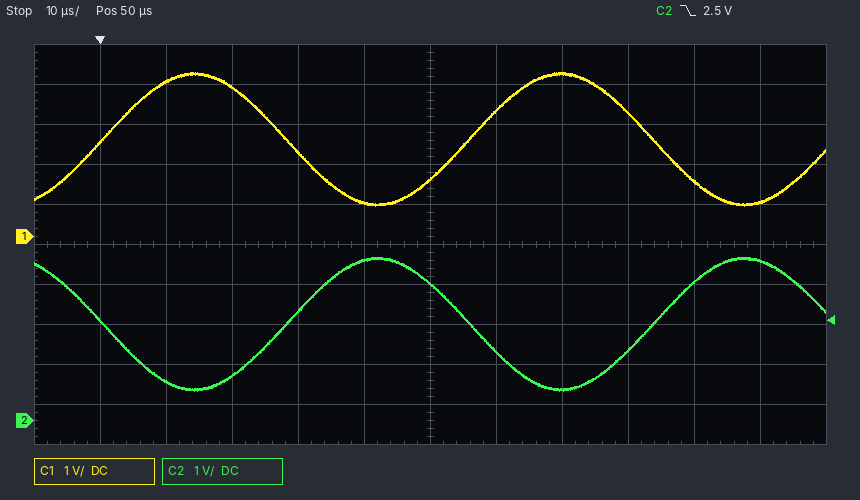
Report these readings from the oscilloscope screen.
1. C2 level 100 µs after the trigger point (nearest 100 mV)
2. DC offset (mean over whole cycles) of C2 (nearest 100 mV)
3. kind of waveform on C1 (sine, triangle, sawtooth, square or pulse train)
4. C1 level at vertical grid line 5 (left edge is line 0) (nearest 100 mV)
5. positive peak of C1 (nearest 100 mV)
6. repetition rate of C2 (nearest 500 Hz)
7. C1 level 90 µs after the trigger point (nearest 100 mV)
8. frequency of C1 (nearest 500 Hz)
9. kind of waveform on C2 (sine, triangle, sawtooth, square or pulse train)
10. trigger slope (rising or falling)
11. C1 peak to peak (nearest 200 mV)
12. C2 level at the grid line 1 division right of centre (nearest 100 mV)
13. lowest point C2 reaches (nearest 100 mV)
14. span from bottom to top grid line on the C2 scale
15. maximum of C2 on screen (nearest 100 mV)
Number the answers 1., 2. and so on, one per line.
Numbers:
1. 4.0 V
2. 2.4 V
3. sine
4. 800 mV
5. 4.1 V
6. 18.0 kHz
7. 1.4 V
8. 18.0 kHz
9. sine
10. falling
11. 3.4 V
12. 1.7 V
13. 700 mV
14. 10 V
15. 4.1 V
